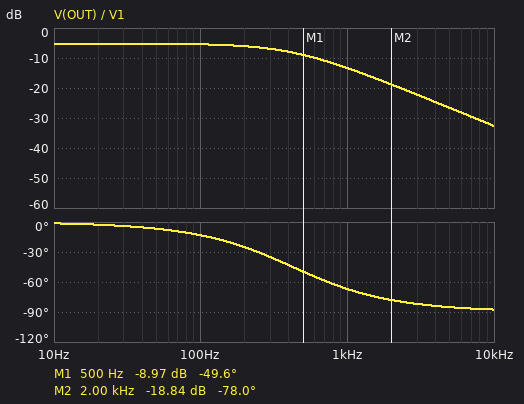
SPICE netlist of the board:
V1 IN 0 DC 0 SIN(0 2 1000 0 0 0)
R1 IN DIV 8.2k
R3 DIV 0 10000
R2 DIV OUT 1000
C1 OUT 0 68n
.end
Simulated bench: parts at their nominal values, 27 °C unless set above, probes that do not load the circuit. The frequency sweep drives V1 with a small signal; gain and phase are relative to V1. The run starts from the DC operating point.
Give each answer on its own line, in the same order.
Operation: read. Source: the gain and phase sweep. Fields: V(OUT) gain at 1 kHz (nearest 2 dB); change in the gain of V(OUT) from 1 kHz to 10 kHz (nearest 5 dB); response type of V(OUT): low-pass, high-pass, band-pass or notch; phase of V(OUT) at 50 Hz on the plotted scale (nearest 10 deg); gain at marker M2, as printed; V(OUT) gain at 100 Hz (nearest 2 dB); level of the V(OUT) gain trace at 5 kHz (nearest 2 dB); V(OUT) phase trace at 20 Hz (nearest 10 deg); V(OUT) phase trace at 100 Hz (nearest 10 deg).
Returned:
-14 dB
-20 dB
low-pass
-10 deg
-18.84 dB
-6 dB
-26 dB
0 deg
-10 deg
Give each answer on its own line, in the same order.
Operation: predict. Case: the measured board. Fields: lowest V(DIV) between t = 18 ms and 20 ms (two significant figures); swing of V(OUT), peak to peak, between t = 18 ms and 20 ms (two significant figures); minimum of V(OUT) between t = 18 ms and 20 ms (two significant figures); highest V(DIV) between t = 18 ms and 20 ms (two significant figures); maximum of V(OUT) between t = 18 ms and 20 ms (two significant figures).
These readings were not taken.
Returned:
-470 mV
860 mV
-430 mV
470 mV
430 mV
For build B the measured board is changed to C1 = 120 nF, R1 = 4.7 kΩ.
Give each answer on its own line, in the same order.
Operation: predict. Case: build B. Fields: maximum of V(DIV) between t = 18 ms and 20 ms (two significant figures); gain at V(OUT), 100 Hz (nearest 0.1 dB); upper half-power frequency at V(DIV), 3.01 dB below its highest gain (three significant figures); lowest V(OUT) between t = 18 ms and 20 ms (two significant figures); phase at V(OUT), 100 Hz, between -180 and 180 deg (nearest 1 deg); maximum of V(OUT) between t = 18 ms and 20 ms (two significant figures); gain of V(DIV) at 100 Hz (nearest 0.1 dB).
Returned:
510 mV
-3.8 dB
336 Hz
-410 mV
-18 deg
410 mV
-3.7 dB
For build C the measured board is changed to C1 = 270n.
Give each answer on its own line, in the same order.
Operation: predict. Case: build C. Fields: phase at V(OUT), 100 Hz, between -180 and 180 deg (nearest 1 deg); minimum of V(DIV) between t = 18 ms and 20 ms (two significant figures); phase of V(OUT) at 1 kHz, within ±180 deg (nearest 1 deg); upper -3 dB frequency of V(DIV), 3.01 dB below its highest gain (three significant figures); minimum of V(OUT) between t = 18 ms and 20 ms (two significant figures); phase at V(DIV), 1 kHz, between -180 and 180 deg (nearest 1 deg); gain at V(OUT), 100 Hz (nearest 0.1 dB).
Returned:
-43 deg
-230 mV
-84 deg
111 Hz
-120 mV
-24 deg
-7.9 dB
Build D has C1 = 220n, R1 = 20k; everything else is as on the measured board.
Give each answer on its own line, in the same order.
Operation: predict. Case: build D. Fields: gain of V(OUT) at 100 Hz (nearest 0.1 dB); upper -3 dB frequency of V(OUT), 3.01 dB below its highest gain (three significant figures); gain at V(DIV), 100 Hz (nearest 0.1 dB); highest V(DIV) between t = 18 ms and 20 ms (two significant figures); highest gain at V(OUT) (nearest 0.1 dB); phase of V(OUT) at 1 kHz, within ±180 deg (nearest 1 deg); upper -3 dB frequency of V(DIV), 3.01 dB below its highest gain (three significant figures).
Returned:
-12.8 dB
94.4 Hz
-12.7 dB
110 mV
-9.5 dB
-85 deg
96.0 Hz
